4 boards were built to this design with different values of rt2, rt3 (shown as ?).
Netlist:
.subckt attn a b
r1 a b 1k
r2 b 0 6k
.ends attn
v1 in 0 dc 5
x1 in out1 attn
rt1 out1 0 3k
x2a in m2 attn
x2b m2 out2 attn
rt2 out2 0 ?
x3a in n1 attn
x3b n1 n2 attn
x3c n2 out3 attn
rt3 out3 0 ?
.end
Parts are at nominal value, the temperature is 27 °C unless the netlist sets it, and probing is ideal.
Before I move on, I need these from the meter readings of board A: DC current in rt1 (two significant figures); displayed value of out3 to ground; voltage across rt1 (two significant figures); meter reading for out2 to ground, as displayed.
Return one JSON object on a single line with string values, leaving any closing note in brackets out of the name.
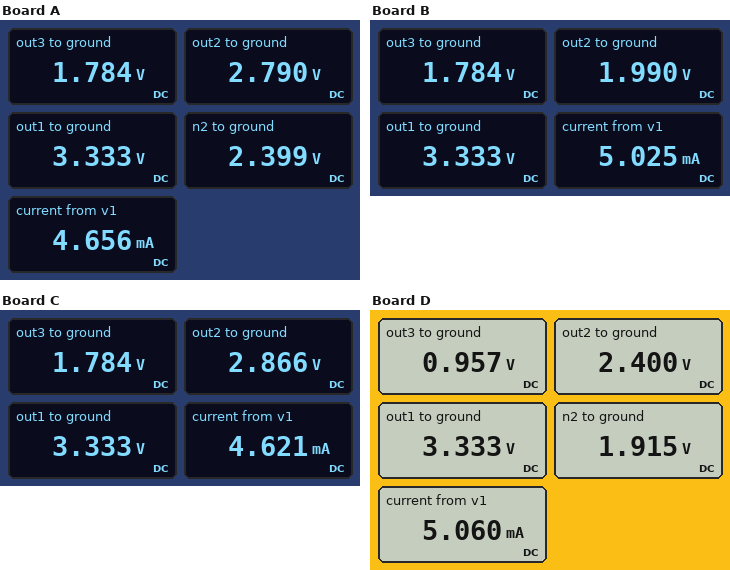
{"DC current in rt1": "1.1 mA", "displayed value of out3 to ground": "1.784 V", "voltage across rt1": "3.3 V", "meter reading for out2 to ground, as displayed": "2.790 V"}
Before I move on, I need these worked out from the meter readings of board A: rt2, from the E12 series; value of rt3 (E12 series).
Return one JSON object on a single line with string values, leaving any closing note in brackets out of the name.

{"rt2, from the E12 series": "8.2 kΩ", "value of rt3": "5.6 kΩ"}
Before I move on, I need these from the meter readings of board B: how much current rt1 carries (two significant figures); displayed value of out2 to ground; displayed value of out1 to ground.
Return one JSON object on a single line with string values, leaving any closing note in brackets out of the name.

{"how much current rt1 carries": "1.1 mA", "displayed value of out2 to ground": "1.990 V", "displayed value of out1 to ground": "3.333 V"}
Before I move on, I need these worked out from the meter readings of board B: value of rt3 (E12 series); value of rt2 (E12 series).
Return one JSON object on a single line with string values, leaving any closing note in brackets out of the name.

{"value of rt3": "5.6 kΩ", "value of rt2": "2.2 kΩ"}
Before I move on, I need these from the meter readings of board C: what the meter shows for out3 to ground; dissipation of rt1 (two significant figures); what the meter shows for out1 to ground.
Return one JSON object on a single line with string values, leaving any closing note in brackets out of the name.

{"what the meter shows for out3 to ground": "1.784 V", "dissipation of rt1": "3.7 mW", "what the meter shows for out1 to ground": "3.333 V"}
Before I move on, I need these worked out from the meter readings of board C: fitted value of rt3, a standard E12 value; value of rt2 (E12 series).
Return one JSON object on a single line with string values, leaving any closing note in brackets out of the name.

{"fitted value of rt3, a standard E12 value": "5.6 kΩ", "value of rt2": "10 kΩ"}
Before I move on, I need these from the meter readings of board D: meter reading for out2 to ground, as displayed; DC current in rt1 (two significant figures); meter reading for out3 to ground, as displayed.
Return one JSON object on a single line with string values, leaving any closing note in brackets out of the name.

{"meter reading for out2 to ground, as displayed": "2.400 V", "DC current in rt1": "1.1 mA", "meter reading for out3 to ground, as displayed": "0.957 V"}
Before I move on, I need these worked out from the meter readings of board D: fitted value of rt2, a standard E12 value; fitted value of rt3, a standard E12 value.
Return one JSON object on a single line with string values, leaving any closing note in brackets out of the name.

{"fitted value of rt2, a standard E12 value": "3.9 kΩ", "fitted value of rt3, a standard E12 value": "1.2 kΩ"}
